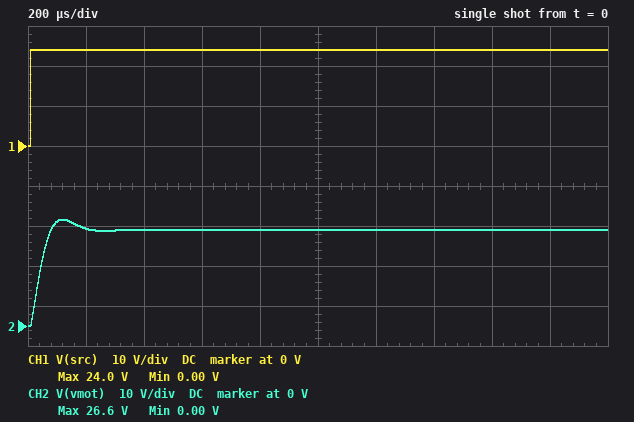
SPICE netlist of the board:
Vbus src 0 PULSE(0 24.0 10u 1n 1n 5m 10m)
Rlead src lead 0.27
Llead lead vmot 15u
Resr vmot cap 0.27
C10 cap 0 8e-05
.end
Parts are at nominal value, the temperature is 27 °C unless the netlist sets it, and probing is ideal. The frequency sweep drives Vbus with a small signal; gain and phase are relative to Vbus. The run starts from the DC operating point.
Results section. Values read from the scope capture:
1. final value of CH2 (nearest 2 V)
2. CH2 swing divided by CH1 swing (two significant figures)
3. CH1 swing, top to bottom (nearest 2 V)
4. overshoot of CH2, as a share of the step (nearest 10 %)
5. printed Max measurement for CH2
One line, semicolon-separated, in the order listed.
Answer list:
24 V; 1.1; 24 V; 10 %; 26.6 V
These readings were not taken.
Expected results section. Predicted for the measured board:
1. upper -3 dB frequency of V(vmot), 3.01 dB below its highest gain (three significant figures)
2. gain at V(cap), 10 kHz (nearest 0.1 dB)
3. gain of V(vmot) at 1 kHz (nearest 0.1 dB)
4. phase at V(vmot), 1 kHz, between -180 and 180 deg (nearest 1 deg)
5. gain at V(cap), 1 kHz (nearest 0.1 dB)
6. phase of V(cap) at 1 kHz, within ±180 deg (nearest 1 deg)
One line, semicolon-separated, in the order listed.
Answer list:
5.73 kHz; -13.3 dB; 0.2 dB; -8 deg; 0.1 dB; -16 deg
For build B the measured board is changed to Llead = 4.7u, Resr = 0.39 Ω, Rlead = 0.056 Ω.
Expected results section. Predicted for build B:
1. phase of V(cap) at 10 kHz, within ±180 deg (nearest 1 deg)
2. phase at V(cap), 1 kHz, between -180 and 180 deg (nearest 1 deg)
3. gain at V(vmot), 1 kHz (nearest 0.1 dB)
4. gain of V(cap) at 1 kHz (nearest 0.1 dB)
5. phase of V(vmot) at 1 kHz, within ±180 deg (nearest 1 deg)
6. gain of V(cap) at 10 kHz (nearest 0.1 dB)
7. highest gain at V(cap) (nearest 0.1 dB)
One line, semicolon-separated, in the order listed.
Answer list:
-102 deg; -13 deg; 0.1 dB; -0.1 dB; -2 deg; -7.2 dB; 0 dB
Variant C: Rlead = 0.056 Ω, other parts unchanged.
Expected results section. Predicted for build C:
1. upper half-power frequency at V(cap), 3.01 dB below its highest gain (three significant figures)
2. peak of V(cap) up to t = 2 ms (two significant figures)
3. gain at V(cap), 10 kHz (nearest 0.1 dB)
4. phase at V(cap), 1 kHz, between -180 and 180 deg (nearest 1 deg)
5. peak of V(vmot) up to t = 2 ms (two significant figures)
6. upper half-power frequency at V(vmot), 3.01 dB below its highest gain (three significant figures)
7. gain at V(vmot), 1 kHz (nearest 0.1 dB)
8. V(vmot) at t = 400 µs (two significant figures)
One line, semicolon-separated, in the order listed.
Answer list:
5.46 kHz; 31 V; -12.2 dB; -10 deg; 32 V; 5.75 kHz; 0.4 dB; 24 V
